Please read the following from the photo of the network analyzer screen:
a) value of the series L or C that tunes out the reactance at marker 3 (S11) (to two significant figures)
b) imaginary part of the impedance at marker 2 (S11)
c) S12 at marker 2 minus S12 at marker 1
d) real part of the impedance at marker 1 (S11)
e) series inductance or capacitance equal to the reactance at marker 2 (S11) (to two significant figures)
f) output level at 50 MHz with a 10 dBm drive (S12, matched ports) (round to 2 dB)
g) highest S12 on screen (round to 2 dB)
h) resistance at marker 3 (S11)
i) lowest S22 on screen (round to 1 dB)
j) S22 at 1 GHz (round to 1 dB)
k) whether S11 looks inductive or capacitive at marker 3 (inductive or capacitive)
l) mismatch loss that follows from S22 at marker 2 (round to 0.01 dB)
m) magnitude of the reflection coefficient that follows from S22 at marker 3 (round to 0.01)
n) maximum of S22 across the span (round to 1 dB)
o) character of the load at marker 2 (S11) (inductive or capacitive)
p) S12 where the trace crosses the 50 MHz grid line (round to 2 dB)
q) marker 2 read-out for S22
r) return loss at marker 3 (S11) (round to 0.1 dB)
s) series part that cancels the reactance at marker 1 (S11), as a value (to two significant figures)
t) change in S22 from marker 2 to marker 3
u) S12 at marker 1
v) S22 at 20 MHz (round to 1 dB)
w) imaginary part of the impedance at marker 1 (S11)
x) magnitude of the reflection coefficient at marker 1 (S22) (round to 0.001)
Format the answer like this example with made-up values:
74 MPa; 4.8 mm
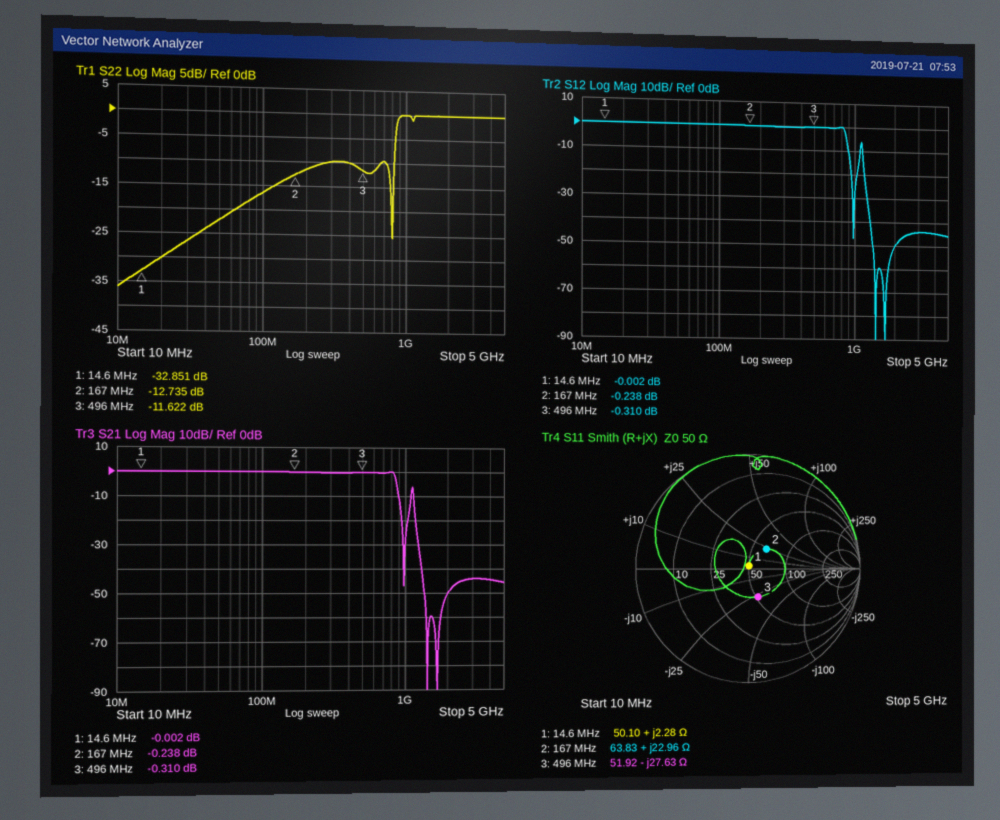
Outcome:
8.9 nH; +22.96 Ω; -0.236 dB; 50.10 Ω; 22 nH; 10 dBm; 0 dB; 51.92 Ω; -36 dB; 0 dB; capacitive; 0.24 dB; 0.26; 0 dB; inductive; 0 dB; -12.735 dB; 11.6 dB; 4.8 nF; 1.113 dB; -0.002 dB; -30 dB; +2.28 Ω; 0.023
